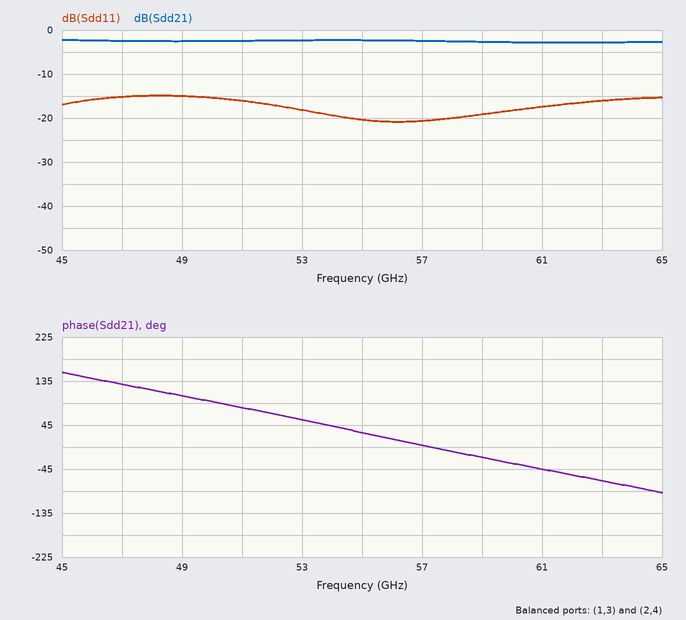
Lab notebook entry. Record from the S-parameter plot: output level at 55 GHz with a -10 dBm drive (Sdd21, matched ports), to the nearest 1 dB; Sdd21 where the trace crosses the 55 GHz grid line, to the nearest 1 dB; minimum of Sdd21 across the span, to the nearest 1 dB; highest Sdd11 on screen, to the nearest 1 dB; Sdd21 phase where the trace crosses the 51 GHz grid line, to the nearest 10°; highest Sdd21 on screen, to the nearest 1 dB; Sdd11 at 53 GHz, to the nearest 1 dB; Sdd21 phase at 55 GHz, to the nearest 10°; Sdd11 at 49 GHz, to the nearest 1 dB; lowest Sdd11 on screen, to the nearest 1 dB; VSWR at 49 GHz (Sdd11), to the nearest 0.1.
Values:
-12 dBm
-2 dB
-3 dB
-15 dB
80°
-2 dB
-18 dB
30°
-15 dB
-21 dB
1.4
